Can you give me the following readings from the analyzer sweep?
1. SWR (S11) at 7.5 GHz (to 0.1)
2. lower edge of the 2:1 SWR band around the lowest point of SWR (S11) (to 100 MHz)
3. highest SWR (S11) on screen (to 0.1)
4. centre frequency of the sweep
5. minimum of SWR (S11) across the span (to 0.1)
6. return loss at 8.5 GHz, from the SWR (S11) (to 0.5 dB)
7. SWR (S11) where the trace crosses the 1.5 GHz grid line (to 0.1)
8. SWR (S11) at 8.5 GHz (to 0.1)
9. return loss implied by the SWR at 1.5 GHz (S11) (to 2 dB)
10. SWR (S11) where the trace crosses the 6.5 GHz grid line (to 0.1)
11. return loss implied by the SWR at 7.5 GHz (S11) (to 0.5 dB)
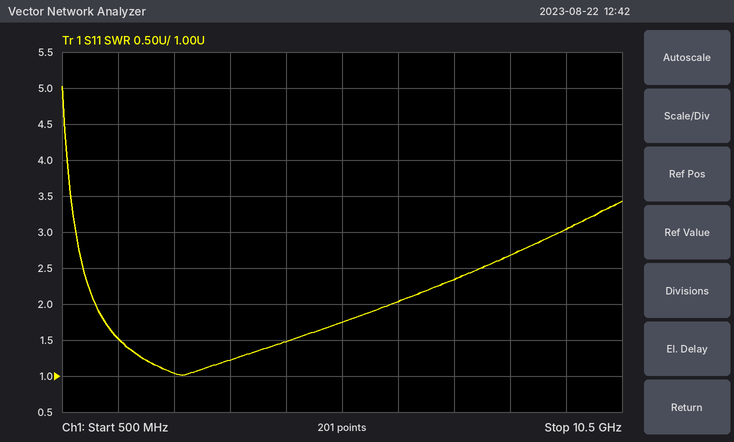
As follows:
2.3
1.1 GHz
5.0
5.5 GHz
1.0
7.0 dB
1.5
2.7
14 dB
2.0
8.0 dB
